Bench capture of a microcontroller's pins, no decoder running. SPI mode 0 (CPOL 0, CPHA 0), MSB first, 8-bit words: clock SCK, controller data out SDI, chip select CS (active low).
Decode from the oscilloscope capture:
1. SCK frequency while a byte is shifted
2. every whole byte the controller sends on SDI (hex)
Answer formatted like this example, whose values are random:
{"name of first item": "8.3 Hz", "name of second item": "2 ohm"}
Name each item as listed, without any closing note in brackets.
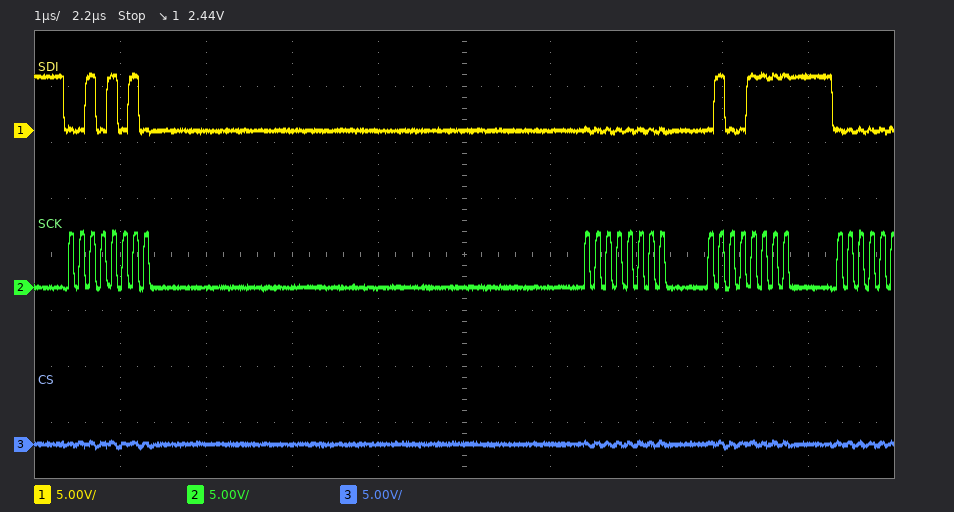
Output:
{"SCK frequency while a byte is shifted": "8 MHz", "every whole byte the controller sends on SDI": "2A 00 4F"}
